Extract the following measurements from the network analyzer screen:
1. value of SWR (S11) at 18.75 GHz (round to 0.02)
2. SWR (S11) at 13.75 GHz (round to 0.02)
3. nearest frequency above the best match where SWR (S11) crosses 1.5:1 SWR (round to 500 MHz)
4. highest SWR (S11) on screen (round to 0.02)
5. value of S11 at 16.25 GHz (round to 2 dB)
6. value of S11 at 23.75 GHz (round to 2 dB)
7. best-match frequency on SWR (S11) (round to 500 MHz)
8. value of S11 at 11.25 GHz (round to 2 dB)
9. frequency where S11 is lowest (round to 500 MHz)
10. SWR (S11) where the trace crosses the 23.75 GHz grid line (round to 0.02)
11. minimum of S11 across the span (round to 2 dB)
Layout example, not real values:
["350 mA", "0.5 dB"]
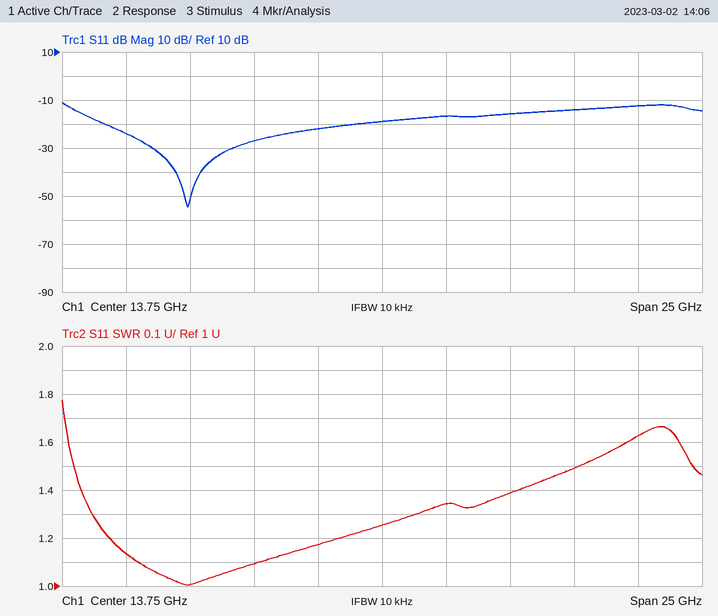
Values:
["1.38", "1.26", "21.5 GHz", "1.78", "-16 dB", "-12 dB", "6.0 GHz", "-22 dB", "6.0 GHz", "1.62", "-54 dB"]
